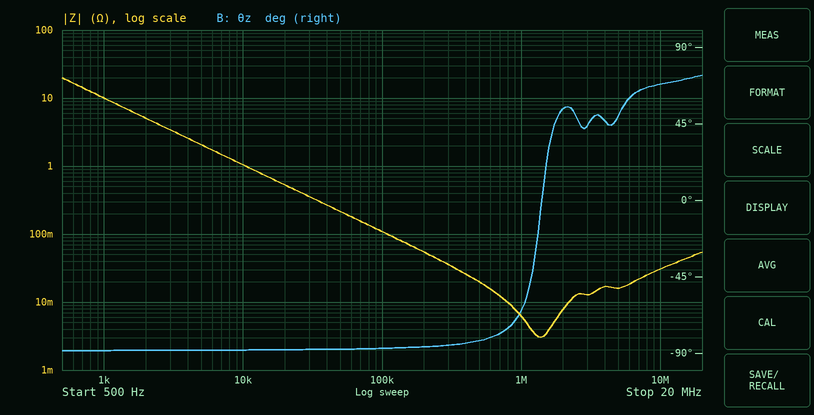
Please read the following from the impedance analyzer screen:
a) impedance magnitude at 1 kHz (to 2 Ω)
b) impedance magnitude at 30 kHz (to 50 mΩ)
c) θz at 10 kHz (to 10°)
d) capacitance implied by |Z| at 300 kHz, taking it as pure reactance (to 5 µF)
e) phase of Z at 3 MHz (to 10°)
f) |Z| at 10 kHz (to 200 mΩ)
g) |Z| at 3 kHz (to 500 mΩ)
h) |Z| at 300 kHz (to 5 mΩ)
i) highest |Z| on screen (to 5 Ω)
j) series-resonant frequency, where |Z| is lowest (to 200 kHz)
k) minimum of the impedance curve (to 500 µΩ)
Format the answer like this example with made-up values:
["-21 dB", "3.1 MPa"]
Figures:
["10 Ω", "350 mΩ", "-90°", "15 µF", "40°", "1.0 Ω", "3.5 Ω", "35 mΩ", "20 Ω", "1.4 MHz", "3.0 mΩ"]
